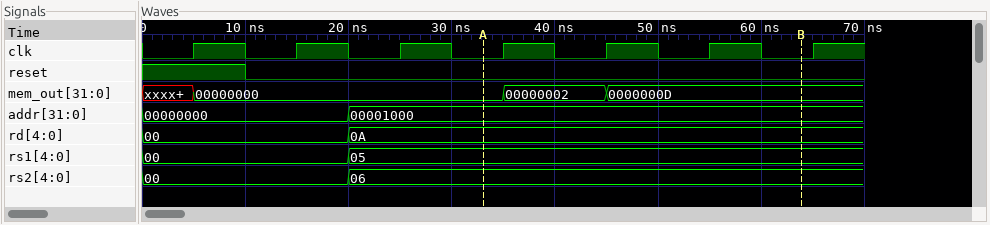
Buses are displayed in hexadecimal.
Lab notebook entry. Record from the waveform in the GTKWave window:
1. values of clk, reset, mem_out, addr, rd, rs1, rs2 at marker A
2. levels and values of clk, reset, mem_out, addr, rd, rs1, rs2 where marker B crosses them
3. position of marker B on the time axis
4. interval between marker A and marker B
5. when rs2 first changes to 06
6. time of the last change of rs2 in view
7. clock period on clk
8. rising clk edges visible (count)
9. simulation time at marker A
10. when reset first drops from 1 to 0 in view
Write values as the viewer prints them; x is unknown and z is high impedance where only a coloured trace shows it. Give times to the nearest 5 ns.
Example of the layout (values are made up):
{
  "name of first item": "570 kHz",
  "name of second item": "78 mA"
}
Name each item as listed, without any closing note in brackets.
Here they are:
{
  "values of clk, reset, mem_out, addr, rd, rs1, rs2 at marker A": "clk=0, reset=0, mem_out=00000000, addr=00001000, rd=0A, rs1=05, rs2=06",
  "levels and values of clk, reset, mem_out, addr, rd, rs1, rs2 where marker B crosses them": "clk=0, reset=0, mem_out=0000000D, addr=00001000, rd=0A, rs1=05, rs2=06",
  "position of marker B on the time axis": "65 ns",
  "interval between marker A and marker B": "30 ns",
  "when rs2 first changes to 06": "20 ns",
  "time of the last change of rs2 in view": "20 ns",
  "clock period on clk": "10 ns",
  "rising clk edges visible": "7",
  "simulation time at marker A": "35 ns",
  "when reset first drops from 1 to 0 in view": "10 ns"
}
